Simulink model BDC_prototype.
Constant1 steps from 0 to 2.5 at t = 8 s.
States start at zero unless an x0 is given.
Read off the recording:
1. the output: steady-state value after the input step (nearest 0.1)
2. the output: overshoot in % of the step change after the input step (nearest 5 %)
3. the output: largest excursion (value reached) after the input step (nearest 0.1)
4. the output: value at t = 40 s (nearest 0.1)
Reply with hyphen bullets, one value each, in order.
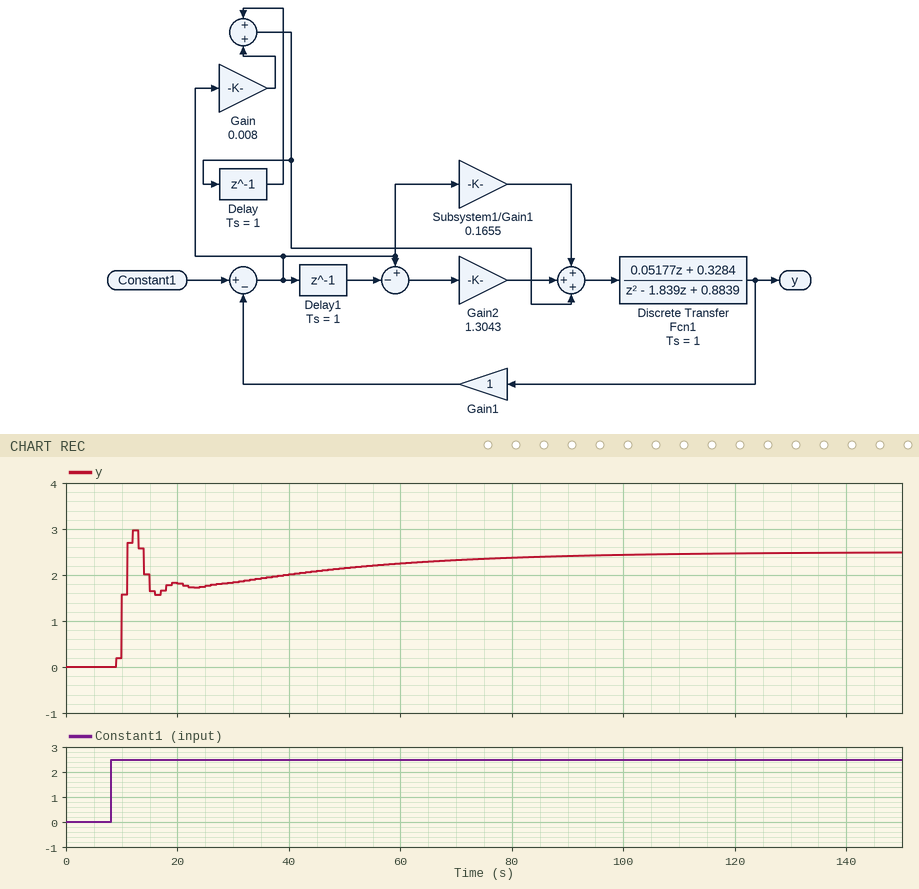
- 2.5
- 20 %
- 3.0
- 2.0
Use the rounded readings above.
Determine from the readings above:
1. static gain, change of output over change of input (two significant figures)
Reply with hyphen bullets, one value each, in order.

- 1.0
